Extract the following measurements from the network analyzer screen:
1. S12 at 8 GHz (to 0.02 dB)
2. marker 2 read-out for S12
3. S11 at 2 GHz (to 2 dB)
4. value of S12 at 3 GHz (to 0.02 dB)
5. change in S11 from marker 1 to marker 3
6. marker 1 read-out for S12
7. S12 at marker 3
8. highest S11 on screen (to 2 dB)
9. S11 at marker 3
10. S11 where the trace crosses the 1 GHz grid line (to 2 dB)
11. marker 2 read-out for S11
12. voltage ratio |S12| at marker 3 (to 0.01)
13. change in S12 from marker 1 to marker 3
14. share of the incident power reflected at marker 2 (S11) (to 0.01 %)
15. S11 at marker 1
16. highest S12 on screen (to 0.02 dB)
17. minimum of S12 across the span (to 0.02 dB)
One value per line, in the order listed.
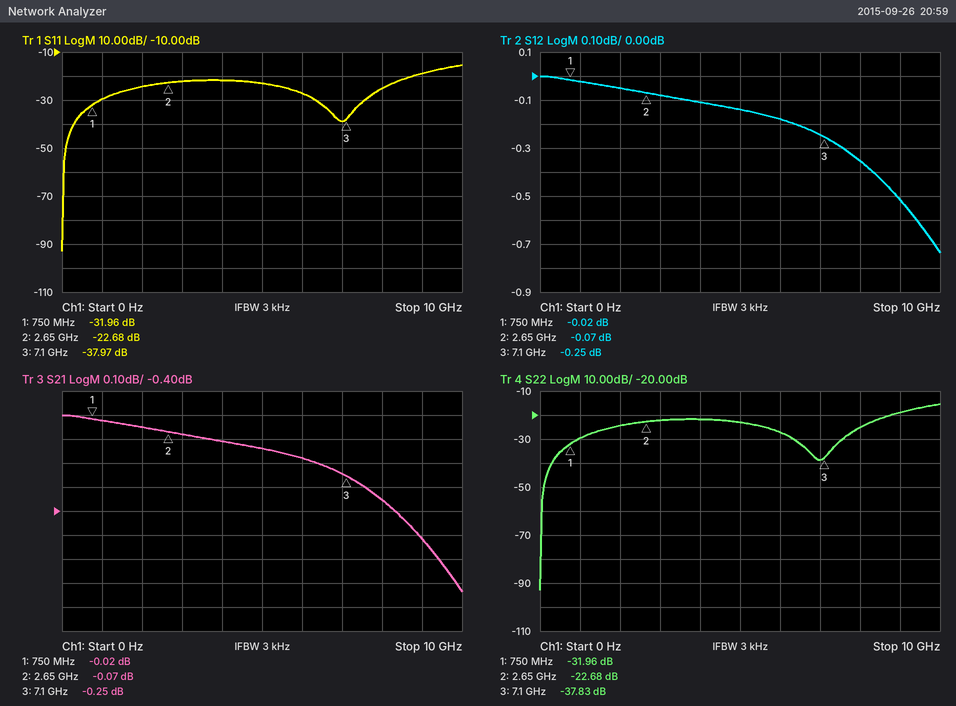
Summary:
-0.36 dB
-0.07 dB
-24 dB
-0.08 dB
-6.01 dB
-0.02 dB
-0.25 dB
-16 dB
-37.97 dB
-30 dB
-22.68 dB
0.97
-0.23 dB
0.54 %
-31.96 dB
0.00 dB
-0.74 dB
